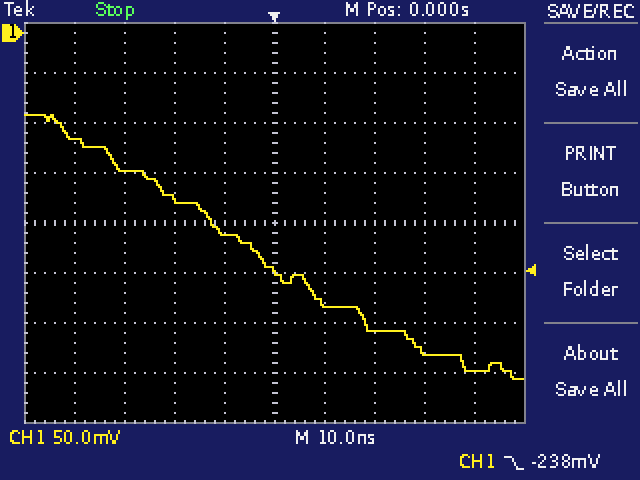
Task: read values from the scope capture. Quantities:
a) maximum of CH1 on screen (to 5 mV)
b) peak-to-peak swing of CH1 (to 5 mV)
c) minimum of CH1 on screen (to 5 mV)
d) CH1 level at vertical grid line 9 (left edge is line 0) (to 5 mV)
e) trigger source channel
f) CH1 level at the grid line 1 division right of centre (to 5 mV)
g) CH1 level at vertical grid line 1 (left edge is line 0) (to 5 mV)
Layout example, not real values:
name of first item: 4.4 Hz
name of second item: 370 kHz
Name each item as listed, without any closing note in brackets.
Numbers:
maximum of CH1 on screen: -80 mV
peak-to-peak swing of CH1: 265 mV
minimum of CH1 on screen: -345 mV
CH1 level at vertical grid line 9 (left edge is line 0): -340 mV
trigger source channel: CH1
CH1 level at the grid line 1 division right of centre: -270 mV
CH1 level at vertical grid line 1 (left edge is line 0): -105 mV
